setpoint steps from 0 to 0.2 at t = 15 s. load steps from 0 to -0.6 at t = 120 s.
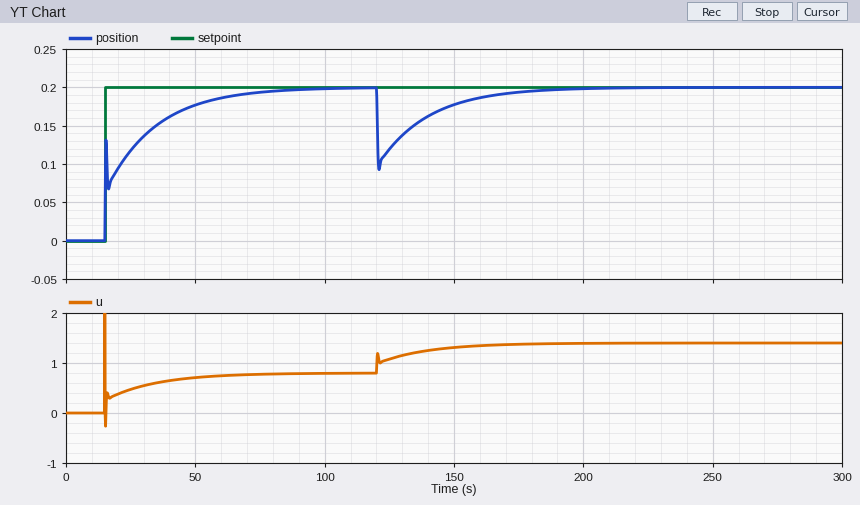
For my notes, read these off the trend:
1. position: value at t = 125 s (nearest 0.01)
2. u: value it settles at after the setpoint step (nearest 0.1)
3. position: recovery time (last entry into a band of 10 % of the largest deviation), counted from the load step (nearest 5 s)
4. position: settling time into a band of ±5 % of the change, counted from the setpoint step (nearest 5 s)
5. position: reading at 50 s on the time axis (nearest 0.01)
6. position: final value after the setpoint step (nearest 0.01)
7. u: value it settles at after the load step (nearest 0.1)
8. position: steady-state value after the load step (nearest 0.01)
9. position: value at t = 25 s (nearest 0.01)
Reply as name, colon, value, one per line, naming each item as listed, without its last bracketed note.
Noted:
position: value at t = 125 s: 0.12
u: value it settles at after the setpoint step: 0.8
position: recovery time (last entry into a band of 10 % of the largest deviation), counted from the load step: 45 s
position: settling time into a band of ±5 % of the change, counted from the setpoint step: 50 s
position: reading at 50 s on the time axis: 0.18
position: final value after the setpoint step: 0.20
u: value it settles at after the load step: 1.4
position: steady-state value after the load step: 0.20
position: value at t = 25 s: 0.12
